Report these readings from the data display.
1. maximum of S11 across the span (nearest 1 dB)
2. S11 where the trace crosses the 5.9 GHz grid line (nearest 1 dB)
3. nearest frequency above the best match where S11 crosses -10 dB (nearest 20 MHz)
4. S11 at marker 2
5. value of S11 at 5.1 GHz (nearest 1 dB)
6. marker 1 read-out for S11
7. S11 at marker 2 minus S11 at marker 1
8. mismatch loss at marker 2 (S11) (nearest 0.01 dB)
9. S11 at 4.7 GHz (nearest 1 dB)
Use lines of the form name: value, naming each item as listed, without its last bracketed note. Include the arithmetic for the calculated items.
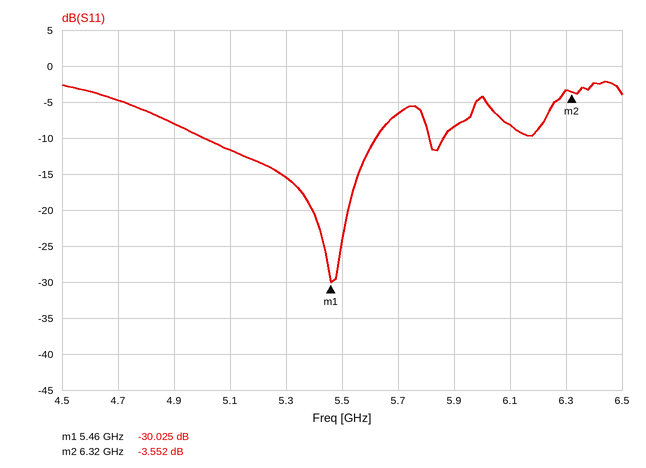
maximum of S11 across the span: -2 dB
S11 where the trace crosses the 5.9 GHz grid line: -8 dB
nearest frequency above the best match where S11 crosses -10 dB: 5.62 GHz
S11 at marker 2: -3.552 dB
value of S11 at 5.1 GHz: -12 dB
marker 1 read-out for S11: -30.025 dB
S11 at marker 2 minus S11 at marker 1: -3.552 − (-30.025) = 26.473 dB
mismatch loss at marker 2 (S11): −10 log10(1 − 10^(-3.552/10)) ≈ 2.53 dB
S11 at 4.7 GHz: -5 dB
